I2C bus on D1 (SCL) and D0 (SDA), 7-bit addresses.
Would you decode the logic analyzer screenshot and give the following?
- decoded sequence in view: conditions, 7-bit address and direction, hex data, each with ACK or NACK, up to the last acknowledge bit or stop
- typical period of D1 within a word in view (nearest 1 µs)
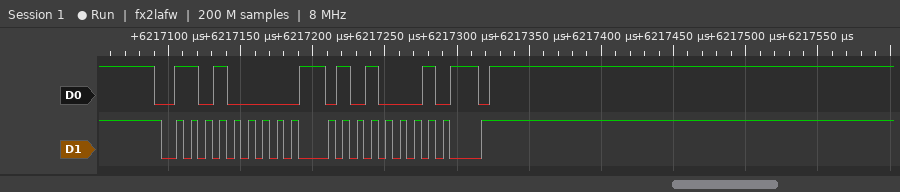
start, address 68 write ACK, 51 ACK, stop
10 µs
